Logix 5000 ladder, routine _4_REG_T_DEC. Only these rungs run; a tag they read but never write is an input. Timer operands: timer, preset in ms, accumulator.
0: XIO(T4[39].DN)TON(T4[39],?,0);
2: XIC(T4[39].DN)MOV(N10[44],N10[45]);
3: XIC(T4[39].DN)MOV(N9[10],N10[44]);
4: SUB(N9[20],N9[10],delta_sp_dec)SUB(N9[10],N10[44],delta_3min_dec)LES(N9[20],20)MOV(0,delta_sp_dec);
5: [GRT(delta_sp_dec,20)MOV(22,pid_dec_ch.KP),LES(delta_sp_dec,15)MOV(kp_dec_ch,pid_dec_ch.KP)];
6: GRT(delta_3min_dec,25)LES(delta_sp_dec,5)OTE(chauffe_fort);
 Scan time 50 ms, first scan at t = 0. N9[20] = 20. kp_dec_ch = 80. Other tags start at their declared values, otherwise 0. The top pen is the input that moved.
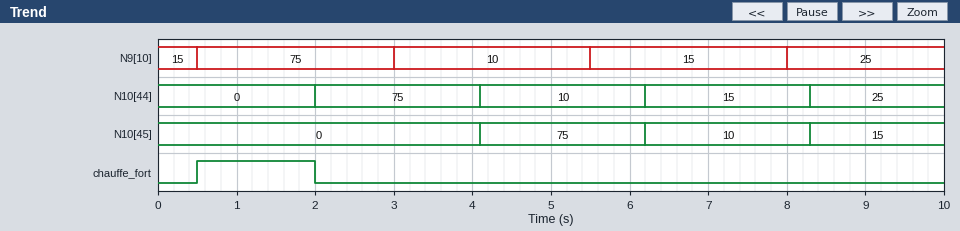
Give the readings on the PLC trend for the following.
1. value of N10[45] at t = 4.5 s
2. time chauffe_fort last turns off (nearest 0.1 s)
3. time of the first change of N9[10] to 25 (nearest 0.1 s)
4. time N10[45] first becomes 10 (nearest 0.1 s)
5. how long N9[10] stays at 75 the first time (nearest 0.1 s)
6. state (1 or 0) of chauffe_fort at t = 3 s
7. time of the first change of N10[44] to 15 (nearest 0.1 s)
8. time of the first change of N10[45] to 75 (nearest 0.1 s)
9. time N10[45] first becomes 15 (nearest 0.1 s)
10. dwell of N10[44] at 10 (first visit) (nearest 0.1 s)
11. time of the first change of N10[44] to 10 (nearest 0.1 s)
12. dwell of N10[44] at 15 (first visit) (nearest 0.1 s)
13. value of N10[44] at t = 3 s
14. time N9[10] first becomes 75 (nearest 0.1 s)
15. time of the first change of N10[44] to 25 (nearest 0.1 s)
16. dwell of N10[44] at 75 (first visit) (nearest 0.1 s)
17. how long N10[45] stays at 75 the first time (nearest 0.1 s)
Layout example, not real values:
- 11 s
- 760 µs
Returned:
- 75
- 2.0 s
- 8.0 s
- 6.2 s
- 2.5 s
- 0
- 6.2 s
- 4.1 s
- 8.3 s
- 2.1 s
- 4.1 s
- 2.1 s
- 75
- 0.5 s
- 8.3 s
- 2.1 s
- 2.1 s
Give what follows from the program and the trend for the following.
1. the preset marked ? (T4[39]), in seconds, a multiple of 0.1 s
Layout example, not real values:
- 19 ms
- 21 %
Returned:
- 2.0 s
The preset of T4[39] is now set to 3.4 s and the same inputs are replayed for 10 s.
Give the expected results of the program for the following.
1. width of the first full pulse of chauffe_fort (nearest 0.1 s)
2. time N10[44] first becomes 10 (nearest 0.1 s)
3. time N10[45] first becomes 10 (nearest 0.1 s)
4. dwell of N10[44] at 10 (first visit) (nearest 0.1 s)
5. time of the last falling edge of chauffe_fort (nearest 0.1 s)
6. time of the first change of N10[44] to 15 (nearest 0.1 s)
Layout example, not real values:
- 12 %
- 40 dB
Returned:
- 2.5 s
- 3.4 s
- 6.9 s
- 3.5 s
- 3.0 s
- 6.9 s
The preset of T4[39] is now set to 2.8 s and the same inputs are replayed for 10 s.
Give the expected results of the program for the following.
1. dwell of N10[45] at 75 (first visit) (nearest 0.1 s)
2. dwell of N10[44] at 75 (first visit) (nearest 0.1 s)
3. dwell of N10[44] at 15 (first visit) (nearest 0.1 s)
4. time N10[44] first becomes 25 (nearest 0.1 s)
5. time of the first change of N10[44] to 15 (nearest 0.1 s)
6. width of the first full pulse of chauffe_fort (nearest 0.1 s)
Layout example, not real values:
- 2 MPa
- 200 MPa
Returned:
- 2.9 s
- 2.9 s
- 2.9 s
- 8.6 s
- 5.7 s
- 2.3 s
